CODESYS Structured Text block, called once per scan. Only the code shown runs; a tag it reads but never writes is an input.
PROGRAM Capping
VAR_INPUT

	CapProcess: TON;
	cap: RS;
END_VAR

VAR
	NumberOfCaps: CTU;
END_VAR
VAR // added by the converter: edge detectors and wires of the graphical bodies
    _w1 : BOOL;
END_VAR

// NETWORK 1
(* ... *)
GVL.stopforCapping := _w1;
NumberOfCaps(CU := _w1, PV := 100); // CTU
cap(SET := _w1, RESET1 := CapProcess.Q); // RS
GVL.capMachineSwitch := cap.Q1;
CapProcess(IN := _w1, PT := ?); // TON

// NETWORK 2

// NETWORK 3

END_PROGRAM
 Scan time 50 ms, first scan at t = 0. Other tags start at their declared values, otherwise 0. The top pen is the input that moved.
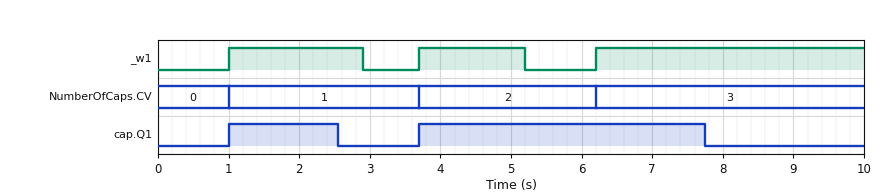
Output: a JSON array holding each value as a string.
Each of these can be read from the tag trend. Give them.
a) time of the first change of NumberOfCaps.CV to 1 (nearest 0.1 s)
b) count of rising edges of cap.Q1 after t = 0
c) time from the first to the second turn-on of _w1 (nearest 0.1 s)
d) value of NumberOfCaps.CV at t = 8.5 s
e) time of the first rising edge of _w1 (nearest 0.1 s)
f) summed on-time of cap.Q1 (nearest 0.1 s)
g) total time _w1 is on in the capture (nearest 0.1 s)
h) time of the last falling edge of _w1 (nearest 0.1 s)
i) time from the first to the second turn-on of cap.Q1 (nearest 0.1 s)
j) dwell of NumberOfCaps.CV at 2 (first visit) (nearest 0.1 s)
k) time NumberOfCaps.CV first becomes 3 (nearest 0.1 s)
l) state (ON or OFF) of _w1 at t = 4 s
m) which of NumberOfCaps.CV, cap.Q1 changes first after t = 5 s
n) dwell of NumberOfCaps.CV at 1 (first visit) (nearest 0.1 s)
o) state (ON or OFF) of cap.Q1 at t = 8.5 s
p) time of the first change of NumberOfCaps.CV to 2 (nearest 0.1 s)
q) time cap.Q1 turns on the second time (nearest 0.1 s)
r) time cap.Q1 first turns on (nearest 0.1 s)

["1.0 s", "2", "2.7 s", "3", "1.0 s", "5.6 s", "7.2 s", "5.2 s", "2.7 s", "2.5 s", "6.2 s", "ON", "NumberOfCaps.CV", "2.7 s", "OFF", "3.7 s", "3.7 s", "1.0 s"]
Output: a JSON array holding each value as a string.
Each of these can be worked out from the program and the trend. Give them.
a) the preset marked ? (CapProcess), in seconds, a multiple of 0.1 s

["1.5 s"]
